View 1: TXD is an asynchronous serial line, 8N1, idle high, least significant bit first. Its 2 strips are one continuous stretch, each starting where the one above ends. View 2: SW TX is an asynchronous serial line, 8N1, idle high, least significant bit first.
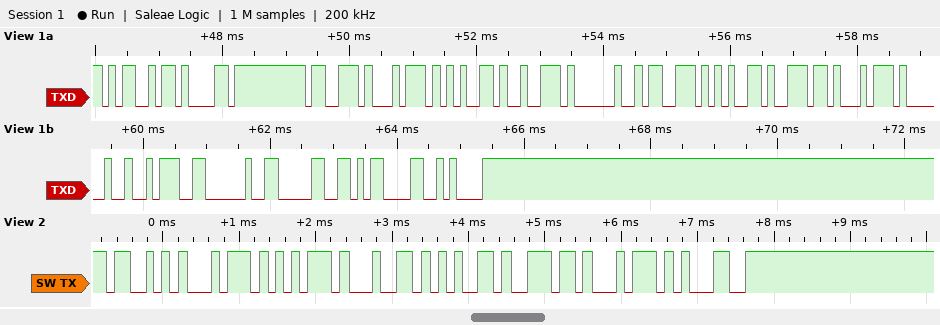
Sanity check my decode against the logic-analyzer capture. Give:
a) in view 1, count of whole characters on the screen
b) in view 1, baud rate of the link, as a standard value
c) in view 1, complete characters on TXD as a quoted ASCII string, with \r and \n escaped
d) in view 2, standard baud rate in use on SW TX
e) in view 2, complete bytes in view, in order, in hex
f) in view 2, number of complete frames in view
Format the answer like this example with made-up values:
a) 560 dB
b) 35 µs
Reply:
a) 17
b) 9600 baud
c) "Master sent : 0\r\n"
d) 9600 baud
e) 0x53 0x74 0x75 0x64 0x65 0x6E 0x74 0x31
f) 8
